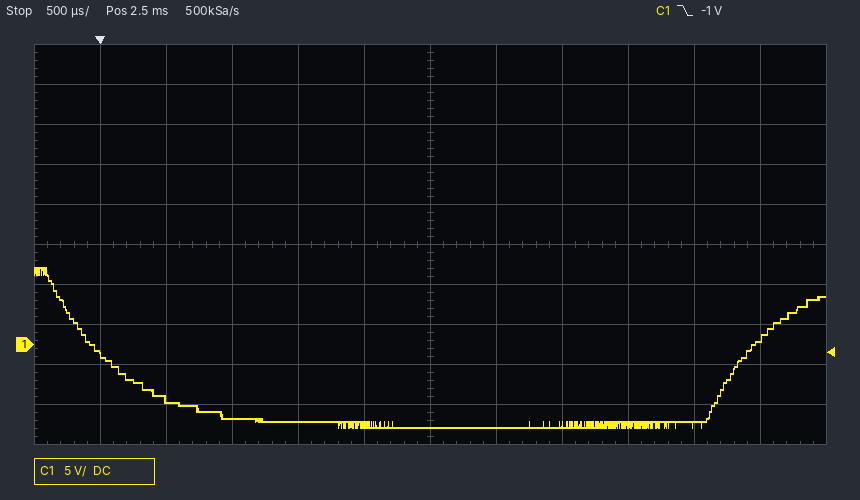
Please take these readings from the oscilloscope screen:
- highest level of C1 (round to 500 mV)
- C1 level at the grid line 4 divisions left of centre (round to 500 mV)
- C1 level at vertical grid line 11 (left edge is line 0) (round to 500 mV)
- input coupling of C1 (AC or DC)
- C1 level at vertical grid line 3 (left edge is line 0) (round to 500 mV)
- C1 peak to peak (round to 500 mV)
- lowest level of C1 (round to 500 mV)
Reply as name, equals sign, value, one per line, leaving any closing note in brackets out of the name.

highest level of C1 = 9.5 V
C1 level at the grid line 4 divisions left of centre = -7.0 V
C1 level at vertical grid line 11 (left edge is line 0) = 1.0 V
input coupling of C1 = DC
C1 level at vertical grid line 3 (left edge is line 0) = -9.0 V
C1 peak to peak = 20.0 V
lowest level of C1 = -10.5 V
